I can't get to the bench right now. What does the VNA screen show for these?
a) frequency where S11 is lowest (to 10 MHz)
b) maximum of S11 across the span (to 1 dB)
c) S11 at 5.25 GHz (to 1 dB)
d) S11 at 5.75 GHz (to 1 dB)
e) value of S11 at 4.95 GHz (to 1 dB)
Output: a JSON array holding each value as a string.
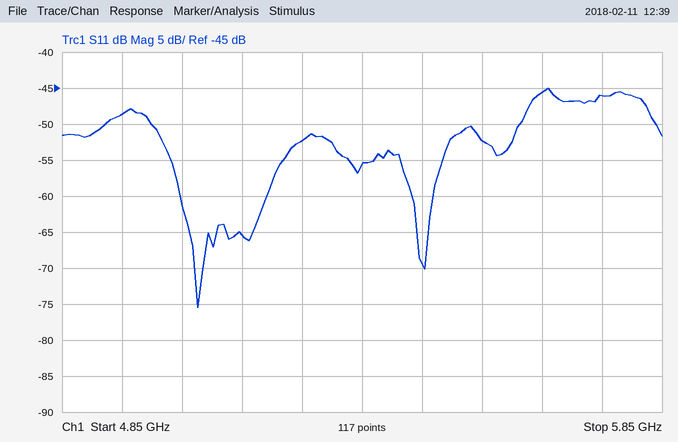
["5.08 GHz", "-45 dB", "-52 dB", "-46 dB", "-49 dB"]
